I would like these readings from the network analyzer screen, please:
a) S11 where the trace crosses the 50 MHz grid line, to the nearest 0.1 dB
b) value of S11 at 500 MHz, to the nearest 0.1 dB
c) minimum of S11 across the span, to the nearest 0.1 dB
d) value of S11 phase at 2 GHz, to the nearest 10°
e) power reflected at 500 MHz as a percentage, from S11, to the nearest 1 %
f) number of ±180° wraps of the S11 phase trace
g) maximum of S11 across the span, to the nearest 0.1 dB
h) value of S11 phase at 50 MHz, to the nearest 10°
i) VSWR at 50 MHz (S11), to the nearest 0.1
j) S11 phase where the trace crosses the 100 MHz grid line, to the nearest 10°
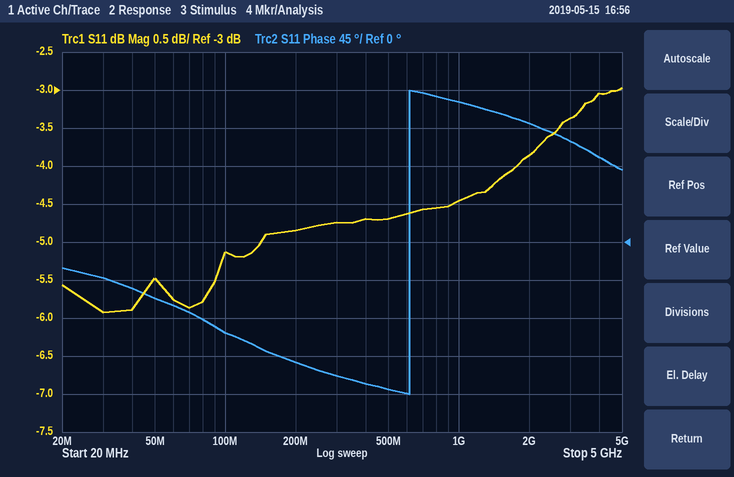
-5.5 dB
-4.7 dB
-5.9 dB
140°
34 %
1
-3.0 dB
-70°
3.3
-110°
